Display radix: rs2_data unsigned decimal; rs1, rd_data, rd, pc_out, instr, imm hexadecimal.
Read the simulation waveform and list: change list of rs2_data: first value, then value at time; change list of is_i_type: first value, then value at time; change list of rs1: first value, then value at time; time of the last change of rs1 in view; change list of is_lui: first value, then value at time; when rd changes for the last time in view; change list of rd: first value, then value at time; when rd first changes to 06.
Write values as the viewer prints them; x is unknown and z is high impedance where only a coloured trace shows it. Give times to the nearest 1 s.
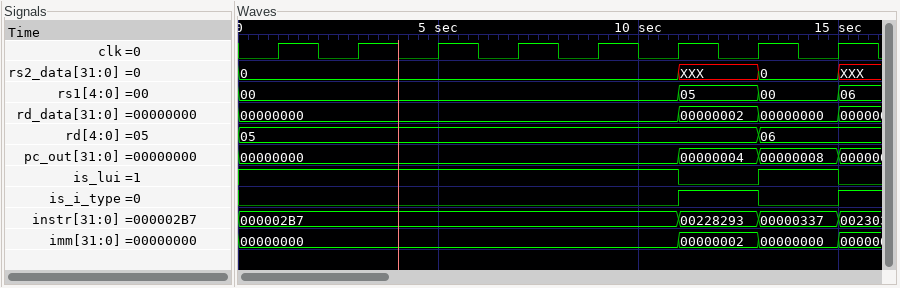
0, XXX at 11 s, 0 at 13 s, XXX at 15 s
0, 1 at 11 s, 0 at 13 s, 1 at 15 s
00, 05 at 11 s, 00 at 13 s, 06 at 15 s
15 s
1, 0 at 11 s, 1 at 13 s, 0 at 15 s
13 s
05, 06 at 13 s
13 s
